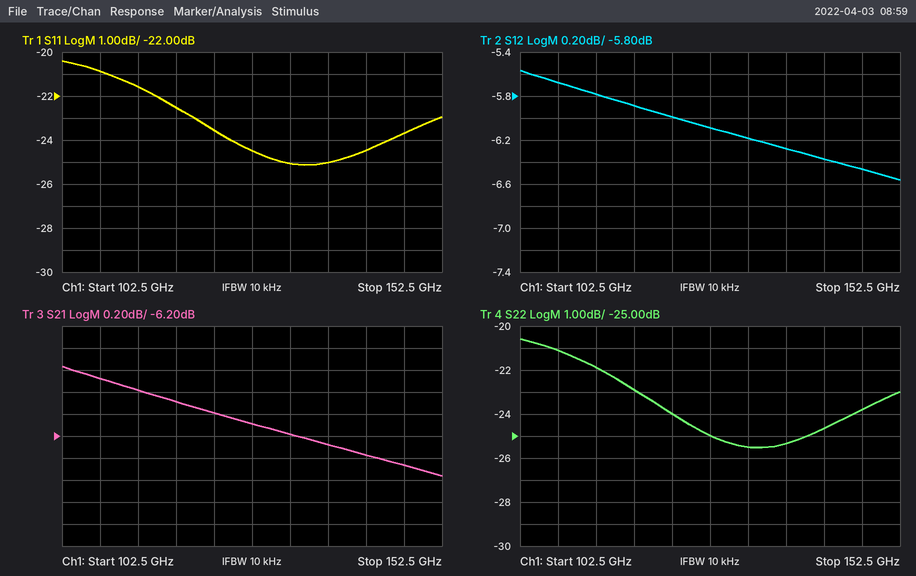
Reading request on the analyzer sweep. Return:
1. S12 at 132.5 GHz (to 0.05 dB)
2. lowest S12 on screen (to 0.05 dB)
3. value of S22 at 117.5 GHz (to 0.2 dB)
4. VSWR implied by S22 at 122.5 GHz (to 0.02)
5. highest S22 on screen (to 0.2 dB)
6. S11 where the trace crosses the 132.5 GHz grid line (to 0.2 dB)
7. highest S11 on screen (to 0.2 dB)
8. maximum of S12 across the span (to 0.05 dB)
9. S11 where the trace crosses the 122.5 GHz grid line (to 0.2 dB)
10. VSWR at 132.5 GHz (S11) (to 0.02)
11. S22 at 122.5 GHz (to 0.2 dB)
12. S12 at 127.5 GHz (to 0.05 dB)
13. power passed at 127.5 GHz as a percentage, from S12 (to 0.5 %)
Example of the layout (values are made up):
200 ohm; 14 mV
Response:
-6.20 dB; -6.55 dB; -22.8 dB; 1.14; -20.6 dB; -25.0 dB; -20.4 dB; -5.55 dB; -23.6 dB; 1.12; -24.0 dB; -6.10 dB; 24.5 %
